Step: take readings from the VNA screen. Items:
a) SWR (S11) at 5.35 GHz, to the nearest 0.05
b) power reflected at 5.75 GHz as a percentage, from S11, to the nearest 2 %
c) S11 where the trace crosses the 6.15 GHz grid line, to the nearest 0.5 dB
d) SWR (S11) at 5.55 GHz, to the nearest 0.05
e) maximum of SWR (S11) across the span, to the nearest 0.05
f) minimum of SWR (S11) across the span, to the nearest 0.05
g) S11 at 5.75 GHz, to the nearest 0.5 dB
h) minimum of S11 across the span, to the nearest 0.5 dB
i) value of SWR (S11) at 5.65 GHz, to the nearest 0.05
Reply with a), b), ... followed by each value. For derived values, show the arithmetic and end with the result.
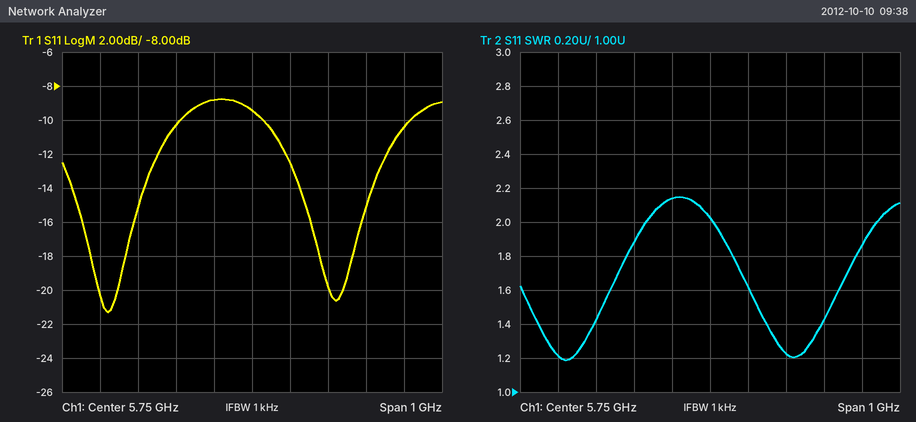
a) 1.20
b) 10^(-9.5/10) ≈ 11.2 %, so 12 % to the nearest 2 %
c) -10.5 dB
d) 1.90
e) 2.15
f) 1.20
g) -9.5 dB
h) -21.5 dB
i) 2.15
